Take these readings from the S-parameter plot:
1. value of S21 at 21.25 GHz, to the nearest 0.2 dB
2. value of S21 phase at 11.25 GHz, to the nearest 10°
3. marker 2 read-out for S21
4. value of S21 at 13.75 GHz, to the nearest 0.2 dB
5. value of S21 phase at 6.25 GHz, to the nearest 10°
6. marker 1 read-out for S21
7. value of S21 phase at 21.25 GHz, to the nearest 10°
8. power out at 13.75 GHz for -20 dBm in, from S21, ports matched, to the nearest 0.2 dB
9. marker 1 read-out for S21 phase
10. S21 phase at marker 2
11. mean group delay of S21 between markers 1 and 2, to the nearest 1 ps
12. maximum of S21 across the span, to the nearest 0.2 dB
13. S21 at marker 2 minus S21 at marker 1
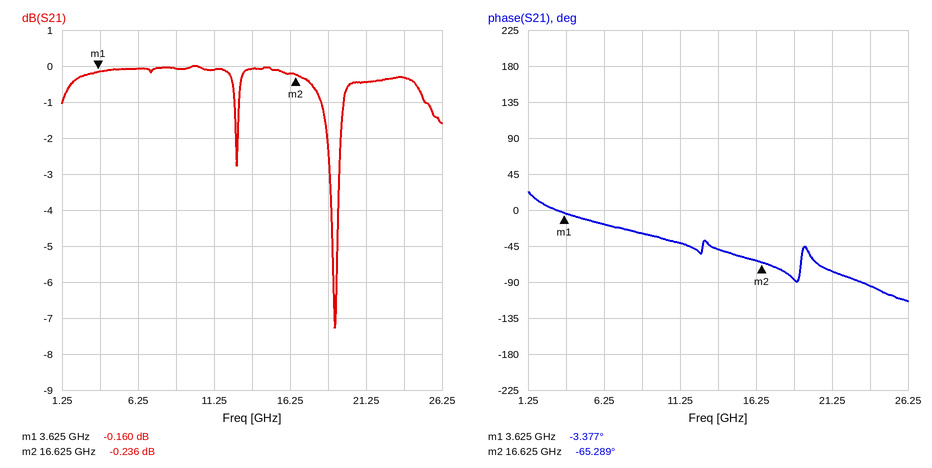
-0.4 dB
-40°
-0.236 dB
0.0 dB
-20°
-0.160 dB
-80°
-20.0 dBm
-3.377°
-65.289°
13 ps
0.0 dB
-0.076 dB
